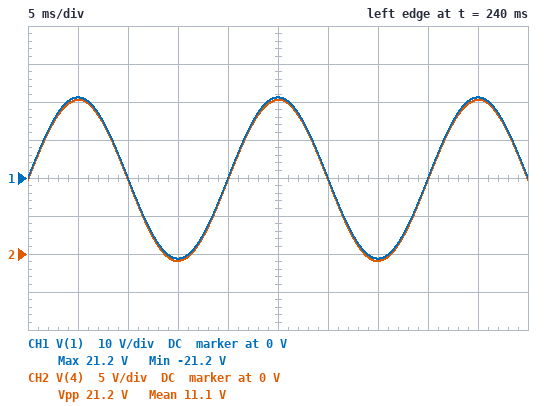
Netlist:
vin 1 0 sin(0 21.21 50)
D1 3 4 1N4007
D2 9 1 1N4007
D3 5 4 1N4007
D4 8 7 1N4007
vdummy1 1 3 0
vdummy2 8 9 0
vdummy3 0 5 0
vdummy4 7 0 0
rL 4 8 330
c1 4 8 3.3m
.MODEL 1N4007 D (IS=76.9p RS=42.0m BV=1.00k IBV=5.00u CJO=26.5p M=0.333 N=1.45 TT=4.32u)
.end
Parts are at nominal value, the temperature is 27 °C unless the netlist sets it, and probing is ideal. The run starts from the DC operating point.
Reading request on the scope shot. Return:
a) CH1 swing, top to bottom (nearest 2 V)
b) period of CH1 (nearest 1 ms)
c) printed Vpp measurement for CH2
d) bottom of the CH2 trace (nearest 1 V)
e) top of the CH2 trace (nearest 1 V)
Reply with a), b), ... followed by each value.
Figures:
a) 42 V
b) 20 ms
c) 21.2 V
d) -1 V
e) 20 V
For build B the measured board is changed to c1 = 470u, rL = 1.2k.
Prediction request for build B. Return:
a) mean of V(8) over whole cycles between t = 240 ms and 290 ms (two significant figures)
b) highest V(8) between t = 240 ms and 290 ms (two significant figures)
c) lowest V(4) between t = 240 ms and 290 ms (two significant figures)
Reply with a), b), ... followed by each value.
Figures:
a) -9.7 V
b) 840 mV
c) -840 mV
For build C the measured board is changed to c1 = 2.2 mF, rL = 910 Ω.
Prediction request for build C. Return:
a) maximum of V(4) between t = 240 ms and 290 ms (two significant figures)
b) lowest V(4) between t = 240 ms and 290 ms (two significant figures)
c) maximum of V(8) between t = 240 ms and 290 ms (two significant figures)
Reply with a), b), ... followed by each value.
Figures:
a) 20 V
b) -860 mV
c) 860 mV
